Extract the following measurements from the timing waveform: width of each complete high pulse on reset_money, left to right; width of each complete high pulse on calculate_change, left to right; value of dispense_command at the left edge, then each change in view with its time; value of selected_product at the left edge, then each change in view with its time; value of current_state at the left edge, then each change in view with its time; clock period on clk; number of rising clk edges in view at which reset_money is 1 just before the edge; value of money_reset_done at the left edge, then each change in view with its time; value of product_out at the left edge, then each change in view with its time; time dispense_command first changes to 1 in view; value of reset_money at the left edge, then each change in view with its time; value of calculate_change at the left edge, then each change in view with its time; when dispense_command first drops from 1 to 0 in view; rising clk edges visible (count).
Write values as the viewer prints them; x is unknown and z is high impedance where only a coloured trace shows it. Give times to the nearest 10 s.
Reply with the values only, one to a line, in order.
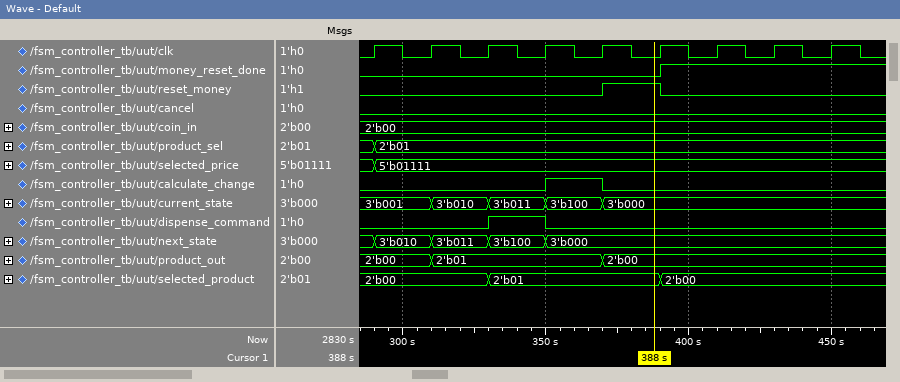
20 s
20 s
0, 1 at 330 s, 0 at 350 s
2'b00, 2'b01 at 330 s, 2'b00 at 390 s
3'b001, 3'b010 at 310 s, 3'b011 at 330 s, 3'b100 at 350 s, 3'b000 at 370 s
20 s
1
0, 1 at 390 s
2'b00, 2'b01 at 310 s, 2'b00 at 370 s
330 s
0, 1 at 370 s, 0 at 390 s
0, 1 at 350 s, 0 at 370 s
350 s
9
